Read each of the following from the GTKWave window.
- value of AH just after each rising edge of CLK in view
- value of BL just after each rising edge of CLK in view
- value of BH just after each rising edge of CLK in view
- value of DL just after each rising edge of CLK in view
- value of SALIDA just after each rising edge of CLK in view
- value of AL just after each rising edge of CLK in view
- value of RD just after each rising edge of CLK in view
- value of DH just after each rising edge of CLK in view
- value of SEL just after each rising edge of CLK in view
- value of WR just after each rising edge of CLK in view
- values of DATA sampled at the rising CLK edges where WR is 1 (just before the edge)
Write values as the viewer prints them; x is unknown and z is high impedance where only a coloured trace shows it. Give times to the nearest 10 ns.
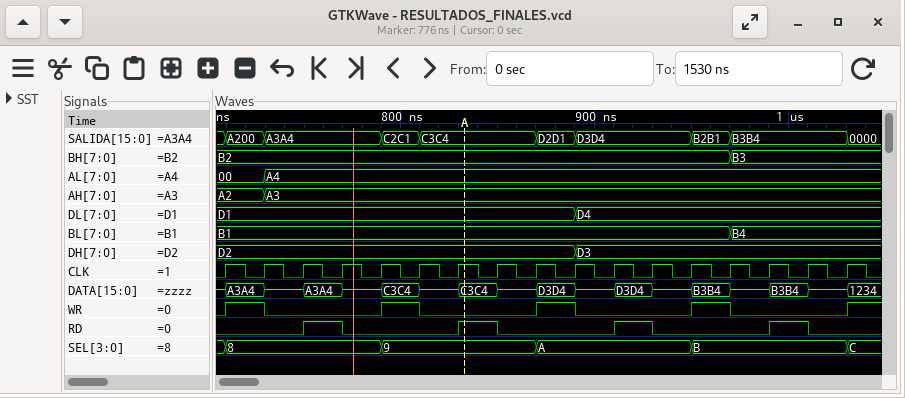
A2, A3, A3, A3, A3, A3, A3, A3, A3, A3, A3, A3, A3, A3, A3, A3, A3
B1, B1, B1, B1, B1, B1, B1, B1, B1, B1, B1, B1, B1, B4, B4, B4, B4
B2, B2, B2, B2, B2, B2, B2, B2, B2, B2, B2, B2, B2, B3, B3, B3, B3
D1, D1, D1, D1, D1, D1, D1, D1, D1, D4, D4, D4, D4, D4, D4, D4, D4
A200, A3A4, A3A4, A3A4, C2C1, C3C4, C3C4, C3C4, D2D1, D3D4, D3D4, D3D4, B2B1, B3B4, B3B4, B3B4, 0000
00, A4, A4, A4, A4, A4, A4, A4, A4, A4, A4, A4, A4, A4, A4, A4, A4
0 0 1 0 0 0 1 0 0 0 1 0 0 0 1 0 0
D2, D2, D2, D2, D2, D2, D2, D2, D2, D3, D3, D3, D3, D3, D3, D3, D3
8, 8, 8, 8, 9, 9, 9, 9, A, A, A, A, B, B, B, B, C
1 0 0 0 1 0 0 0 1 0 0 0 1 0 0 0 1
A3A4, C3C4, D3D4, B3B4
